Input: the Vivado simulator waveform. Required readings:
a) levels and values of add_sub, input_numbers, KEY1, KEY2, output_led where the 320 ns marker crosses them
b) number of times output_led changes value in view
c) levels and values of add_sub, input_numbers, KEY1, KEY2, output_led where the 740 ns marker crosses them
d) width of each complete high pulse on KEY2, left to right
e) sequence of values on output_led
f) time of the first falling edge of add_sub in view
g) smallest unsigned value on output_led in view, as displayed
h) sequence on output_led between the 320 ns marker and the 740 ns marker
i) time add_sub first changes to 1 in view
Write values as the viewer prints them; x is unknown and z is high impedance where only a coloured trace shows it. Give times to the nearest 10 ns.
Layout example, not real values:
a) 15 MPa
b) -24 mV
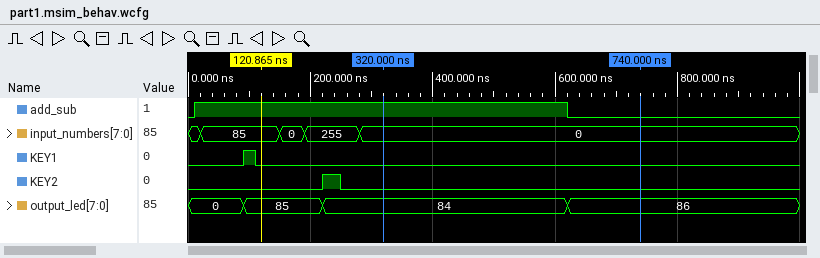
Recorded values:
a) add_sub=1, input_numbers=0, KEY1=0, KEY2=0, output_led=84
b) 3
c) add_sub=0, input_numbers=0, KEY1=0, KEY2=0, output_led=86
d) 30 ns
e) 0, 85, 84, 86
f) 620 ns
g) 0
h) 84, 86
i) 10 ns
